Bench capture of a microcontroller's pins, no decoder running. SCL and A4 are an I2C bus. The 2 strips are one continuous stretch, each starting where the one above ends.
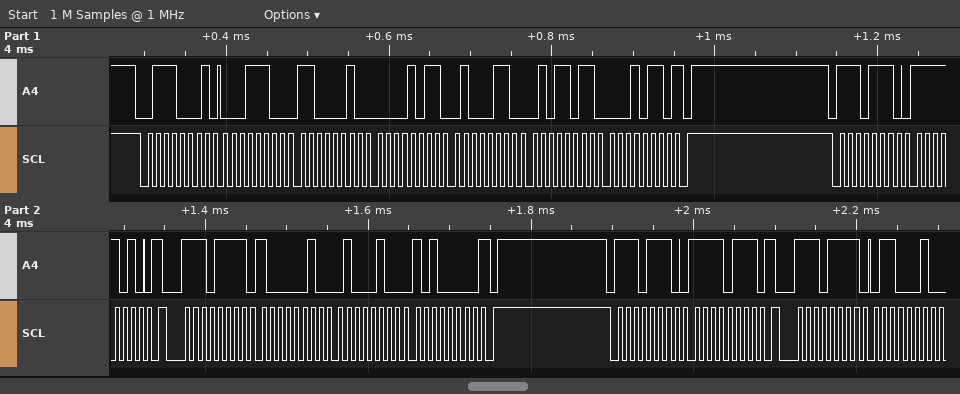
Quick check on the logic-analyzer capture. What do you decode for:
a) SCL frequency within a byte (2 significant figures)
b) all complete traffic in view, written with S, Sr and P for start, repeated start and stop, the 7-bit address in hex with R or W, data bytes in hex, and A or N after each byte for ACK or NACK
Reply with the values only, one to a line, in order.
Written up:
100 kHz
S 38R A 1C A C2 A 0B A 46 A 5B A 16 N P S 77W A FA A Sr 77R A 82 A 44 A A0 N P S 77W A F7 A Sr 77R A 62 A
